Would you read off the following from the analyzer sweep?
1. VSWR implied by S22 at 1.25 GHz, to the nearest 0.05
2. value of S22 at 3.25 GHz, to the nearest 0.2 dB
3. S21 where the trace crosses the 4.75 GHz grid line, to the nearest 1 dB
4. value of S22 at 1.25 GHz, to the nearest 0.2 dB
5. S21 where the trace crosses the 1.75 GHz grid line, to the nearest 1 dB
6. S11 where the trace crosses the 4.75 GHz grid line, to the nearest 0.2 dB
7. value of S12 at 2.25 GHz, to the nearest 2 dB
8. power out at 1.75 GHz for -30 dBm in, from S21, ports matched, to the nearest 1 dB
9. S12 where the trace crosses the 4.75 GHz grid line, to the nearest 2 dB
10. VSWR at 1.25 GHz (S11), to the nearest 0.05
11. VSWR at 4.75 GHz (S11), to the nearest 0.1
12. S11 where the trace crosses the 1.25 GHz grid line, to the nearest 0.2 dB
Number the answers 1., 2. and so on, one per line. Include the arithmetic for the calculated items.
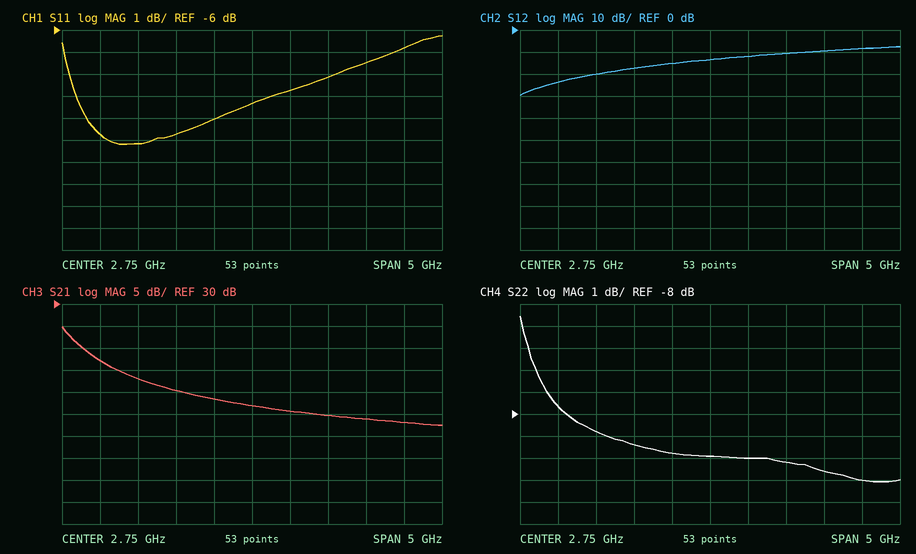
1. |Γ| = 10^(-8.8/20) = 0.3631; VSWR = (1 + 0.3631)/(1 − 0.3631) ≈ 2.14, so 2.15 to the nearest 0.05
2. -10.0 dB
3. 3 dB
4. -8.8 dB
5. 10 dB
6. -6.8 dB
7. -16 dB
8. -30 dBm + (10 dB) = -20 dBm
9. -8 dB
10. |Γ| = 10^(-11.2/20) = 0.2754; VSWR = (1 + 0.2754)/(1 − 0.2754) ≈ 1.76, so 1.75 to the nearest 0.05
11. |Γ| = 10^(-6.8/20) = 0.4571; VSWR = (1 + 0.4571)/(1 − 0.4571) ≈ 2.7
12. -11.2 dB
